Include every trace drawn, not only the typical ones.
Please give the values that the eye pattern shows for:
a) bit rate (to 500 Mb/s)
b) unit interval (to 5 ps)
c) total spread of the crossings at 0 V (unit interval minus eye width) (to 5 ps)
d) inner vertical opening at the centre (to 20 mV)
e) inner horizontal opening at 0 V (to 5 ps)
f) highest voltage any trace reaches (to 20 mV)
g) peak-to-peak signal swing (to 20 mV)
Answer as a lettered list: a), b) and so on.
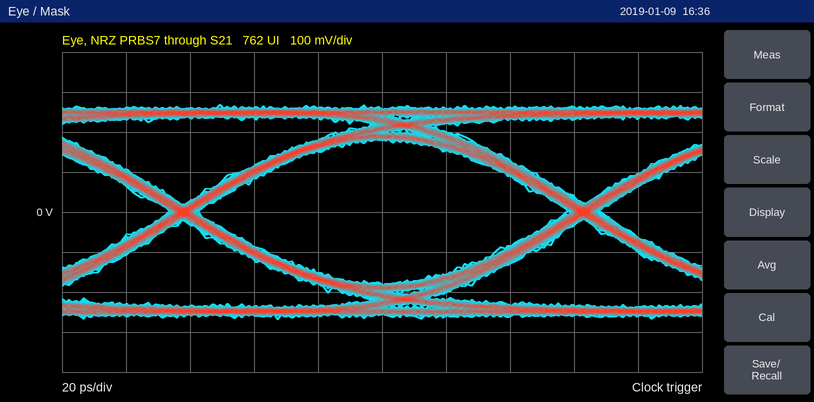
a) 8.0 Gb/s
b) 125 ps
c) 10 ps
d) 360 mV
e) 115 ps
f) 260 mV
g) 540 mV
